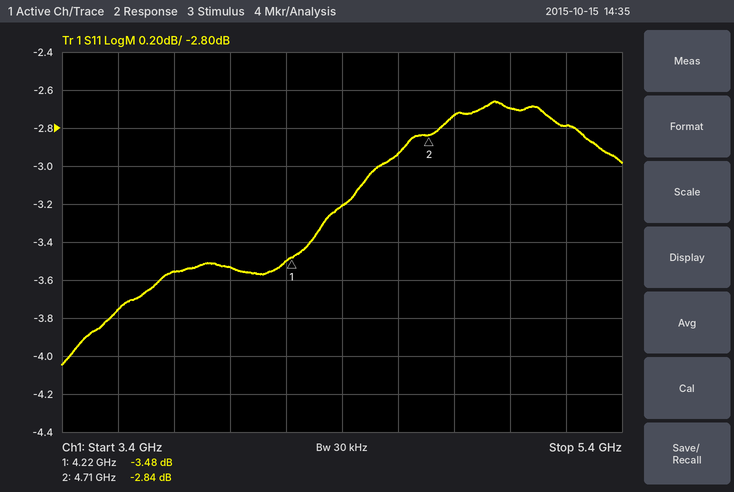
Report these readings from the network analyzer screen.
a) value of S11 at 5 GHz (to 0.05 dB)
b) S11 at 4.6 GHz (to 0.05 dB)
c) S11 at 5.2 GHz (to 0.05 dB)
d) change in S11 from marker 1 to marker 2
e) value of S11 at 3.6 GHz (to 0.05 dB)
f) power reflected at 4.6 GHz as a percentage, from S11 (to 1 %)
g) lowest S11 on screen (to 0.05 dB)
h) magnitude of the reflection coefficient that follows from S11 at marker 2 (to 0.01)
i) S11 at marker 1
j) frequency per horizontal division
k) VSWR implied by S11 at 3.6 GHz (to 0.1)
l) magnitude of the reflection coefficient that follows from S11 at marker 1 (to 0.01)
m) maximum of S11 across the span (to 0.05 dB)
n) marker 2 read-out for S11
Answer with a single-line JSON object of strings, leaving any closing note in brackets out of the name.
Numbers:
{"value of S11 at 5 GHz": "-2.70 dB", "S11 at 4.6 GHz": "-2.95 dB", "S11 at 5.2 GHz": "-2.80 dB", "change in S11 from marker 1 to marker 2": "0.64 dB", "value of S11 at 3.6 GHz": "-3.75 dB", "power reflected at 4.6 GHz as a percentage, from S11": "51 %", "lowest S11 on screen": "-4.05 dB", "magnitude of the reflection coefficient that follows from S11 at marker 2": "0.72", "S11 at marker 1": "-3.48 dB", "frequency per horizontal division": "200 MHz", "VSWR implied by S11 at 3.6 GHz": "4.7", "magnitude of the reflection coefficient that follows from S11 at marker 1": "0.67", "maximum of S11 across the span": "-2.65 dB", "marker 2 read-out for S11": "-2.84 dB"}
